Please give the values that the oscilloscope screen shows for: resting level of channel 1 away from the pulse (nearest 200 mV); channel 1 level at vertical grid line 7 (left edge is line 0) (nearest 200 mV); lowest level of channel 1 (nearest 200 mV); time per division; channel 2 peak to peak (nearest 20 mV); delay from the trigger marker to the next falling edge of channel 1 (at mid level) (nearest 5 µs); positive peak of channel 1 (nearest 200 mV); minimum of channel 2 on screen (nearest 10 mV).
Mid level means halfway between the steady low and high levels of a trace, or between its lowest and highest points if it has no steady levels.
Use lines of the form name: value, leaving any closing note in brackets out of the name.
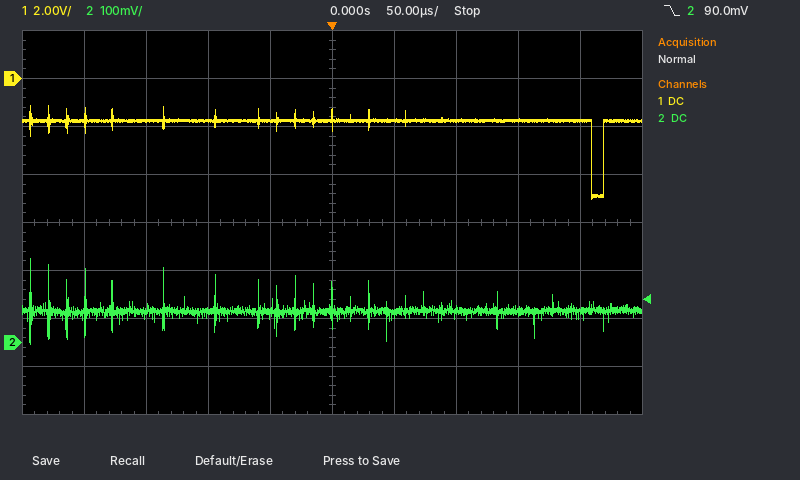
resting level of channel 1 away from the pulse: -1.8 V
channel 1 level at vertical grid line 7 (left edge is line 0): -1.8 V
lowest level of channel 1: -5.0 V
time per division: 50 µs
channel 2 peak to peak: 180 mV
delay from the trigger marker to the next falling edge of channel 1 (at mid level): 210 µs
positive peak of channel 1: -1.2 V
minimum of channel 2 on screen: 0 mV
